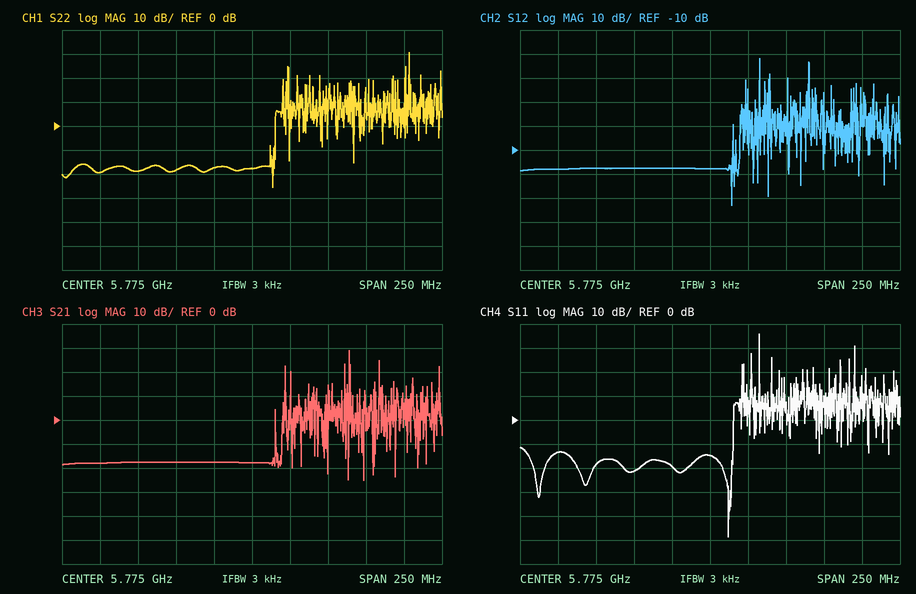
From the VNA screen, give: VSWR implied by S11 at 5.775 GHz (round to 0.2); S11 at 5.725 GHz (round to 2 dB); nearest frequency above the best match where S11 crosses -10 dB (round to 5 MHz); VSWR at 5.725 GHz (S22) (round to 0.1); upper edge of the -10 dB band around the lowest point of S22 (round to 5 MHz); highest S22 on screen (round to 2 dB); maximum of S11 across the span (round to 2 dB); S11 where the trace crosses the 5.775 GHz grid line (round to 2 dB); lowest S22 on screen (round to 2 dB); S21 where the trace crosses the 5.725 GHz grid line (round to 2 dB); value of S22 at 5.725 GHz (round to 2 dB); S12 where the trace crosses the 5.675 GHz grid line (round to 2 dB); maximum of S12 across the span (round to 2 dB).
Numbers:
1.4
-22 dB
5.790 GHz
1.3
5.790 GHz
30 dB
36 dB
-14 dB
-26 dB
-18 dB
-18 dB
-18 dB
28 dB
